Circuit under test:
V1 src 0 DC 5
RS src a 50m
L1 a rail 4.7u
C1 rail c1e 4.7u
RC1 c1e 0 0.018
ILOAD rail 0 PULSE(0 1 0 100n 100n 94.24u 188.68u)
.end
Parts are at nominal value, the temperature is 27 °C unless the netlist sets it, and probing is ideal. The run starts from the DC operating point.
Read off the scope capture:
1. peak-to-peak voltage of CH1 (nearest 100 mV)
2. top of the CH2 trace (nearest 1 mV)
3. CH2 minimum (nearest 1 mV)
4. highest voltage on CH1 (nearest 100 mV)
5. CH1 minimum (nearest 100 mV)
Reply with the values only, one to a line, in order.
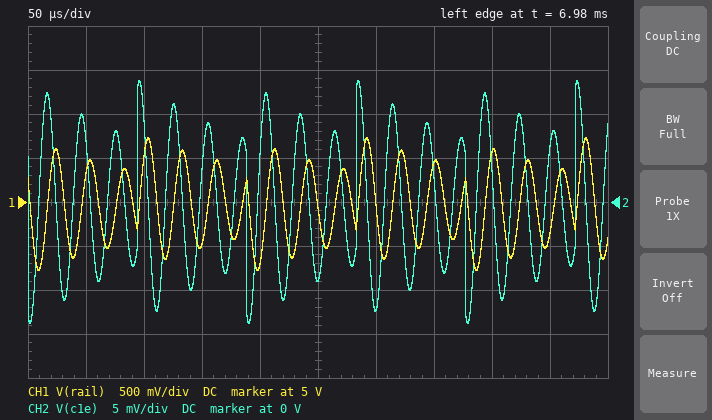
1.5 V
14 mV
-14 mV
5.7 V
4.2 V
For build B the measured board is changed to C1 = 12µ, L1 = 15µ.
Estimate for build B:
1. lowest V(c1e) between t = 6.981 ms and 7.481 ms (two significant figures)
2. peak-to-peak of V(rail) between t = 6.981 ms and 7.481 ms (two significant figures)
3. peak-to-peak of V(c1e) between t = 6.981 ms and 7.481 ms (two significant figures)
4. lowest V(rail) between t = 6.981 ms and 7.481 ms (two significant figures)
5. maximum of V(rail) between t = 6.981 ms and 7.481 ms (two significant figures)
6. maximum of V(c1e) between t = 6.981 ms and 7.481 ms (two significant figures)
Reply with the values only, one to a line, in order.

-11 mV
1.3 V
21 mV
4.3 V
5.6 V
11 mV
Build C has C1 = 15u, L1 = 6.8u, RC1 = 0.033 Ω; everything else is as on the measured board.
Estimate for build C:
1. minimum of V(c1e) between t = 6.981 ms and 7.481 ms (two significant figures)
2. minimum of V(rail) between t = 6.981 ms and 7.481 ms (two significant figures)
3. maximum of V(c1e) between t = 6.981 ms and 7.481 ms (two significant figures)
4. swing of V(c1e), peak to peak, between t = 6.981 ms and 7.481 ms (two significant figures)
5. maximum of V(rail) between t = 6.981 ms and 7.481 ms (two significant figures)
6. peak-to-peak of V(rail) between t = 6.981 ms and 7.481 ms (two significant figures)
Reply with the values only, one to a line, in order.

-74 mV
3.6 V
74 mV
150 mV
6.4 V
2.8 V
